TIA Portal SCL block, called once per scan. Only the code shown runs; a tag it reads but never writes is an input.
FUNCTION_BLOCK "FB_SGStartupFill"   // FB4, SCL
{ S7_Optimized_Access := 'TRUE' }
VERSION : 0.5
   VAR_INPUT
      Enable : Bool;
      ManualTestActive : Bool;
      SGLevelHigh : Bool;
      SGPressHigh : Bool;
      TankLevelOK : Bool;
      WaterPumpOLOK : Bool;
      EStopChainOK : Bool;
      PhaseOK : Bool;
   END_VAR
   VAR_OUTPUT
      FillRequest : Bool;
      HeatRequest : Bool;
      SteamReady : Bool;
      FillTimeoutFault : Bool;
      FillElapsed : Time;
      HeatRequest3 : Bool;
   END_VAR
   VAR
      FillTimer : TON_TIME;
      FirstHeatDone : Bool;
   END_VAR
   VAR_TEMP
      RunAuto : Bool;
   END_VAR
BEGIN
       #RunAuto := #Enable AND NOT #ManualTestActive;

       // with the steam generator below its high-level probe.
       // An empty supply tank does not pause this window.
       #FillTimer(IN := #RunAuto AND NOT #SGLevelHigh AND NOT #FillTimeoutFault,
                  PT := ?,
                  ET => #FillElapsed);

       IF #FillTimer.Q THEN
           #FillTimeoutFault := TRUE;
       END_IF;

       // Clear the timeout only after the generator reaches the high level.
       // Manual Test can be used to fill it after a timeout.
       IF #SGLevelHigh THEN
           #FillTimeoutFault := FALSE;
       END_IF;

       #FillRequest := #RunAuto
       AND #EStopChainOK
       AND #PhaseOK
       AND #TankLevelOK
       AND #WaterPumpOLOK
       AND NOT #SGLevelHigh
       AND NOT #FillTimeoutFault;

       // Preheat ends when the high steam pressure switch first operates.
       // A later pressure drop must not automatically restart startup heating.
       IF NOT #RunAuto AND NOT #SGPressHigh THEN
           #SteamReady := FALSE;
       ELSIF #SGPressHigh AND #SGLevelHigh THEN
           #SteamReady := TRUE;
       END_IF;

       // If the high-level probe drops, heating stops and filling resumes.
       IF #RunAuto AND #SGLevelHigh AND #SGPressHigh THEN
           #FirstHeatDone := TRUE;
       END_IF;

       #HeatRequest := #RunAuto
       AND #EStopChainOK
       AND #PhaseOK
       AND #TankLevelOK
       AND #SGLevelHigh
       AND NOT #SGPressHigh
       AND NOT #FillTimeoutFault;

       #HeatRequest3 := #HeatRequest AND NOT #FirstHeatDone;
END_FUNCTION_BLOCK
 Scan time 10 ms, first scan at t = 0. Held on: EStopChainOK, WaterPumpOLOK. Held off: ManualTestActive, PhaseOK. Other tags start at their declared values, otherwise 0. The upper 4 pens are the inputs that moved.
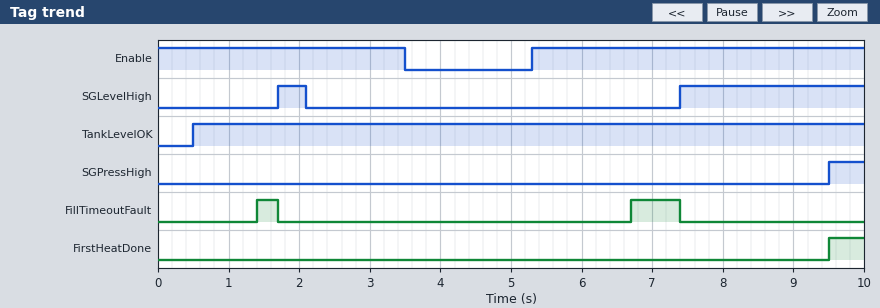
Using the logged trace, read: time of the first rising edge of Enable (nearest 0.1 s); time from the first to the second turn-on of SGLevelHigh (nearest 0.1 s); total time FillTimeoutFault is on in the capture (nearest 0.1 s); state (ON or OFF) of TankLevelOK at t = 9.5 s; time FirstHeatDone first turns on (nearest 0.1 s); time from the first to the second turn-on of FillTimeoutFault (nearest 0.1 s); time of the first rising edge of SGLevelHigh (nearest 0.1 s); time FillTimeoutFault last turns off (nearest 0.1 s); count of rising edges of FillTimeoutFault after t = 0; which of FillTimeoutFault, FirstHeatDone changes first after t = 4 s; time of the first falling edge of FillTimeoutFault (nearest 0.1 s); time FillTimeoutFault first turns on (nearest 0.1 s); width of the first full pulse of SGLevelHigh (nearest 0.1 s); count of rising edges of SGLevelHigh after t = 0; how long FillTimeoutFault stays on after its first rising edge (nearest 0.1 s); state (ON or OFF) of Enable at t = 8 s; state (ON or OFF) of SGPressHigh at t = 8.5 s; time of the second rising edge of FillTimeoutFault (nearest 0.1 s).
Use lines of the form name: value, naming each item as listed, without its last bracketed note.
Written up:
time of the first rising edge of Enable: 5.3 s
time from the first to the second turn-on of SGLevelHigh: 5.7 s
total time FillTimeoutFault is on in the capture: 1.0 s
state (ON or OFF) of TankLevelOK at t = 9.5 s: ON
time FirstHeatDone first turns on: 9.5 s
time from the first to the second turn-on of FillTimeoutFault: 5.3 s
time of the first rising edge of SGLevelHigh: 1.7 s
time FillTimeoutFault last turns off: 7.4 s
count of rising edges of FillTimeoutFault after t = 0: 2
which of FillTimeoutFault, FirstHeatDone changes first after t = 4 s: FillTimeoutFault
time of the first falling edge of FillTimeoutFault: 1.7 s
time FillTimeoutFault first turns on: 1.4 s
width of the first full pulse of SGLevelHigh: 0.4 s
count of rising edges of SGLevelHigh after t = 0: 2
how long FillTimeoutFault stays on after its first rising edge: 0.3 s
state (ON or OFF) of Enable at t = 8 s: ON
state (ON or OFF) of SGPressHigh at t = 8.5 s: OFF
time of the second rising edge of FillTimeoutFault: 6.7 s
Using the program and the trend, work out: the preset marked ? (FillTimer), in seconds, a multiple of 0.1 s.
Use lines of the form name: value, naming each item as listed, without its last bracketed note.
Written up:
the preset marked ? (FillTimer), in seconds, a multiple of 0.1 s: 1.4 s
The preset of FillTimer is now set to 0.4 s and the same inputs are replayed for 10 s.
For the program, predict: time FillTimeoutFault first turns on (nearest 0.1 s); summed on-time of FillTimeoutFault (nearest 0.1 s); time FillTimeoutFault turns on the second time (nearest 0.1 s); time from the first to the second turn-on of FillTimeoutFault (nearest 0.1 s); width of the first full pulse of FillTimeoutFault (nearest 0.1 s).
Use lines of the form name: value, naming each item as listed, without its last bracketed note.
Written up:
time FillTimeoutFault first turns on: 0.4 s
summed on-time of FillTimeoutFault: 6.2 s
time FillTimeoutFault turns on the second time: 2.5 s
time from the first to the second turn-on of FillTimeoutFault: 2.1 s
width of the first full pulse of FillTimeoutFault: 1.3 s
